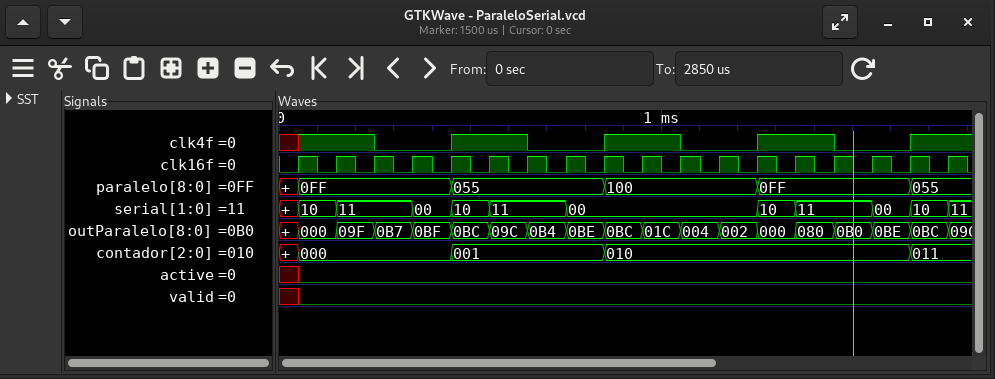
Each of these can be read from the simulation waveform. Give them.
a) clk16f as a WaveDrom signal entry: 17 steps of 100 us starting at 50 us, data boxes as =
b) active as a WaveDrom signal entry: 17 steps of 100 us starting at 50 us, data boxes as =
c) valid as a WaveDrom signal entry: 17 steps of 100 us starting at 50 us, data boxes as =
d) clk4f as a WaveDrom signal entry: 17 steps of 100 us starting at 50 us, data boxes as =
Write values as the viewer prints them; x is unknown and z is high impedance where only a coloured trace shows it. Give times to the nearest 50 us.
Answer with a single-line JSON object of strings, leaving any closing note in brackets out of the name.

{"clk16f as a WaveDrom signal entry: 17 steps of 100 us starting at 50 us, data boxes as =": "{name: 'clk16f', wave: 'p................'}", "active as a WaveDrom signal entry: 17 steps of 100 us starting at 50 us, data boxes as =": "{name: 'active', wave: '0................'}", "valid as a WaveDrom signal entry: 17 steps of 100 us starting at 50 us, data boxes as =": "{name: 'valid', wave: '0................'}", "clk4f as a WaveDrom signal entry: 17 steps of 100 us starting at 50 us, data boxes as =": "{name: 'clk4f', wave: '1.0.1.0.1.0.1.0.1'}"}
